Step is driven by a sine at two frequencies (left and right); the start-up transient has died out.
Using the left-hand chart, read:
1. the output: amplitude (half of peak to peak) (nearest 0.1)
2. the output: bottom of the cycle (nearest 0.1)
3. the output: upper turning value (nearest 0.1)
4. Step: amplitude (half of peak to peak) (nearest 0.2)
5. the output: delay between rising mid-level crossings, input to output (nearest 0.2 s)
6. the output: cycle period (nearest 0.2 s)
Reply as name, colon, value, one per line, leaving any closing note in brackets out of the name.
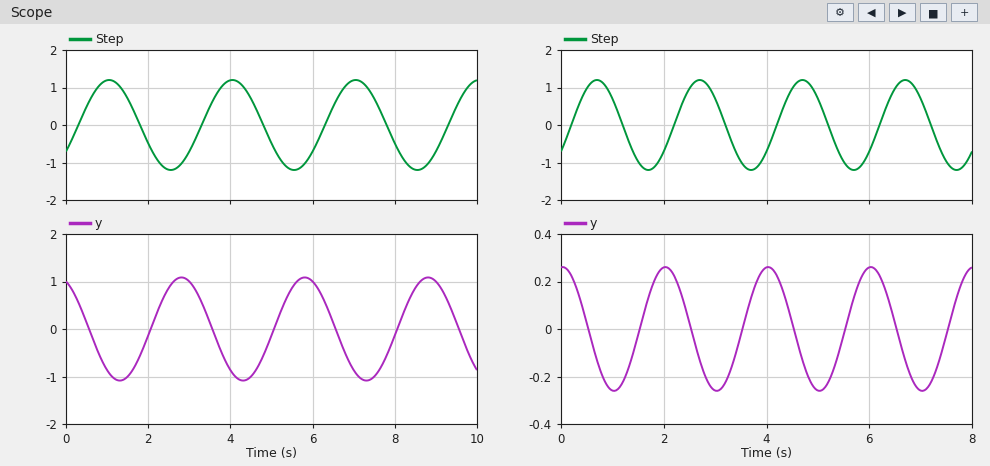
the output: amplitude (half of peak to peak): 1.1
the output: bottom of the cycle: -1.1
the output: upper turning value: 1.1
Step: amplitude (half of peak to peak): 1.2
the output: delay between rising mid-level crossings, input to output: 1.8 s
the output: cycle period: 3.0 s
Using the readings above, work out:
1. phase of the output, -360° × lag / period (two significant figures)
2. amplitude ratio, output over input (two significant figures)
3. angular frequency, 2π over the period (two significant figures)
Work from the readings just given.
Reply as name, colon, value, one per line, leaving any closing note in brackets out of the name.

phase of the output, -360° × lag / period: -220°
amplitude ratio, output over input: 0.92
angular frequency, 2π over the period: 2.1 rad/s
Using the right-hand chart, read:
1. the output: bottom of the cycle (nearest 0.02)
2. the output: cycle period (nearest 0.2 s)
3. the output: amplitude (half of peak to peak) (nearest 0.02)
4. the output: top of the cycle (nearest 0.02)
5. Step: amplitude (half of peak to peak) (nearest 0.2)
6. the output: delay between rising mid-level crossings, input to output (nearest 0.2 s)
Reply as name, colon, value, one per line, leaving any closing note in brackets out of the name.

the output: bottom of the cycle: -0.26
the output: cycle period: 2.0 s
the output: amplitude (half of peak to peak): 0.26
the output: top of the cycle: 0.26
Step: amplitude (half of peak to peak): 1.2
the output: delay between rising mid-level crossings, input to output: 1.4 s
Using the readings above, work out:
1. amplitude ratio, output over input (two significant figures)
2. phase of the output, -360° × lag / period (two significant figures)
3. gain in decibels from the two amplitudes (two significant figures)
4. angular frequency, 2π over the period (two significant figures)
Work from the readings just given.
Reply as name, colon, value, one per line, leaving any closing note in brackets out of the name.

amplitude ratio, output over input: 0.22
phase of the output, -360° × lag / period: -250°
gain in decibels from the two amplitudes: -13 dB
angular frequency, 2π over the period: 3.1 rad/s
